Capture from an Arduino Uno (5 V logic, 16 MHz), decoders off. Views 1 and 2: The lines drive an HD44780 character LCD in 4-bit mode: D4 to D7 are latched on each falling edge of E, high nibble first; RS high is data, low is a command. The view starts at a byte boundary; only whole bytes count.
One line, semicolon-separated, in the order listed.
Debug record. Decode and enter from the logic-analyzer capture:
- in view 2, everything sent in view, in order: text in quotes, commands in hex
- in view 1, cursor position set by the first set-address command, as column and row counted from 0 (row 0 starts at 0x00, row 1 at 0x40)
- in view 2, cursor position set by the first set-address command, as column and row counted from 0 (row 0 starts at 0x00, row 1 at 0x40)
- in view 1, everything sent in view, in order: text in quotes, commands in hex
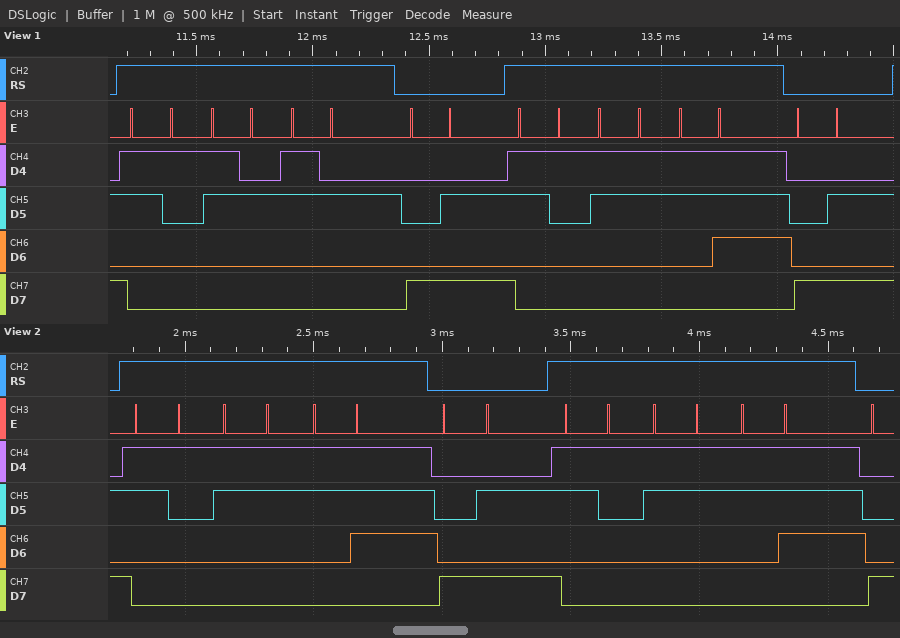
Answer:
"137" 0x8A "137"; column 10, row 0; column 10, row 0; "122" 0x8A "137" 0x8A
